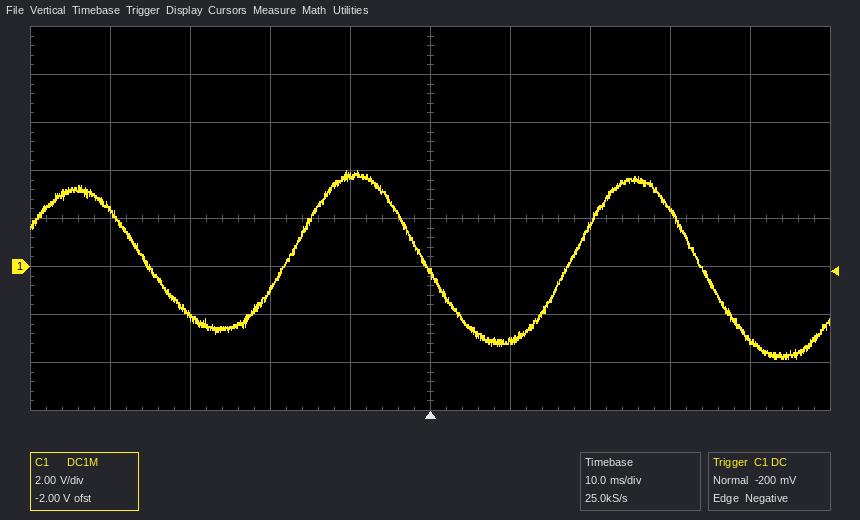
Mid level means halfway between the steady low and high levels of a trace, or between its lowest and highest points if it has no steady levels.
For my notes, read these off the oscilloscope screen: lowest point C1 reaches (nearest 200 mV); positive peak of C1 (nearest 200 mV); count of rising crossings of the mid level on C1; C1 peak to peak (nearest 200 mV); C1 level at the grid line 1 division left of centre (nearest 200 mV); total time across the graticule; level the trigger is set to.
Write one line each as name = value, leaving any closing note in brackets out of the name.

lowest point C1 reaches = -3.8 V
positive peak of C1 = 4.0 V
count of rising crossings of the mid level on C1 = 2
C1 peak to peak = 7.8 V
C1 level at the grid line 1 division left of centre = 3.8 V
total time across the graticule = 100 ms
level the trigger is set to = -200 mV
